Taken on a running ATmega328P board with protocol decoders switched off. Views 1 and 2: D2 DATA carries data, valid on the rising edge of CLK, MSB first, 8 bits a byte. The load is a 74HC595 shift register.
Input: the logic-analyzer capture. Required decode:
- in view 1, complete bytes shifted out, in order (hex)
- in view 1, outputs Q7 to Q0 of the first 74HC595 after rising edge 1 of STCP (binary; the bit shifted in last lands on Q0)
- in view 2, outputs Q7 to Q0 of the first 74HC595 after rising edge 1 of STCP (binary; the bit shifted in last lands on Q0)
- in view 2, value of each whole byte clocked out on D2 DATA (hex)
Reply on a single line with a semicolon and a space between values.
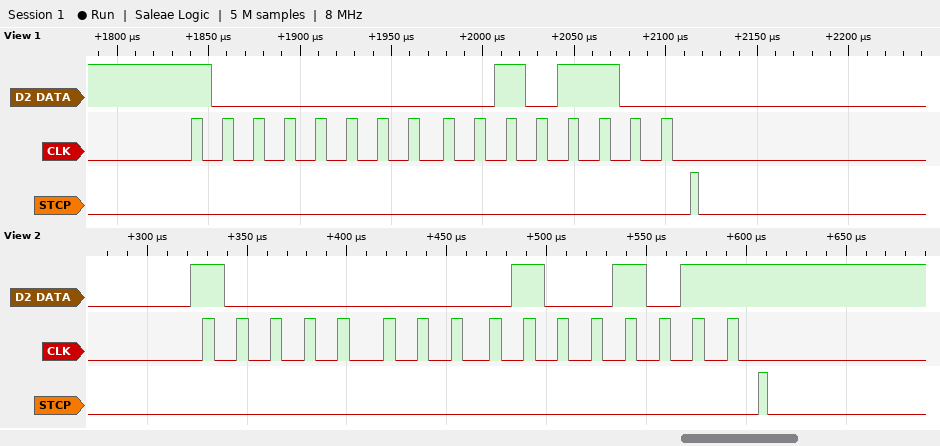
0x80 0x2C; 00101100; 01001011; 80 4B
